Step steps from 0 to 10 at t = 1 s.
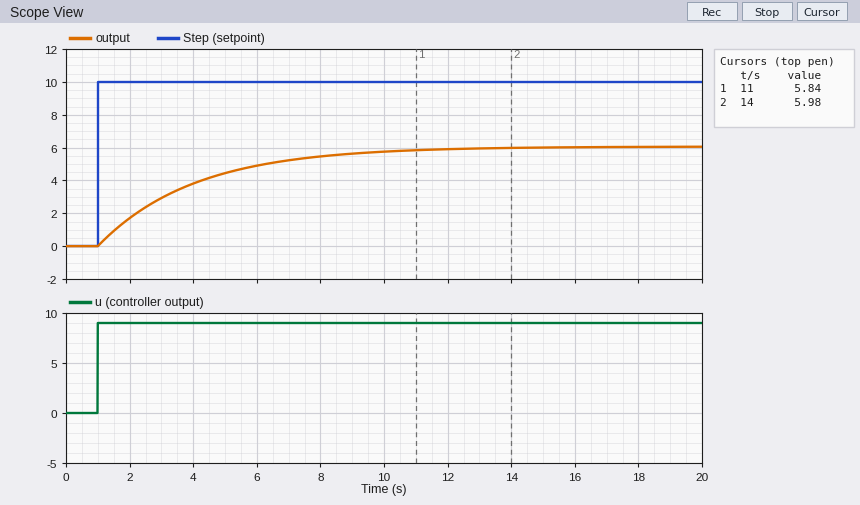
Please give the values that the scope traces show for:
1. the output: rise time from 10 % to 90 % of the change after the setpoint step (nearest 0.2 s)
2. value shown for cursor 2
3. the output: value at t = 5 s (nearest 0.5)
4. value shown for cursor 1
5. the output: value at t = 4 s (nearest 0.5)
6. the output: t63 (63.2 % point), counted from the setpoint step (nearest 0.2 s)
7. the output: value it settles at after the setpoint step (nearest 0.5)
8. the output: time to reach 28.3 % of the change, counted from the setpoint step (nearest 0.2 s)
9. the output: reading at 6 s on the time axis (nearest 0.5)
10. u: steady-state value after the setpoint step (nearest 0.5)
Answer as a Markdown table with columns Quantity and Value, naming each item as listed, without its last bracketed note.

| Quantity | Value |
|---|---|
| the output: rise time from 10 % to 90 % of the change after the setpoint step | 6.6 s |
| value shown for cursor 2 | 5.98 |
| the output: value at t = 5 s | 4.5 |
| value shown for cursor 1 | 5.84 |
| the output: value at t = 4 s | 4.0 |
| the output: t63 (63.2 % point), counted from the setpoint step | 3.0 s |
| the output: value it settles at after the setpoint step | 6.0 |
| the output: time to reach 28.3 % of the change, counted from the setpoint step | 1.0 s |
| the output: reading at 6 s on the time axis | 5.0 |
| u: steady-state value after the setpoint step | 9.0 |
